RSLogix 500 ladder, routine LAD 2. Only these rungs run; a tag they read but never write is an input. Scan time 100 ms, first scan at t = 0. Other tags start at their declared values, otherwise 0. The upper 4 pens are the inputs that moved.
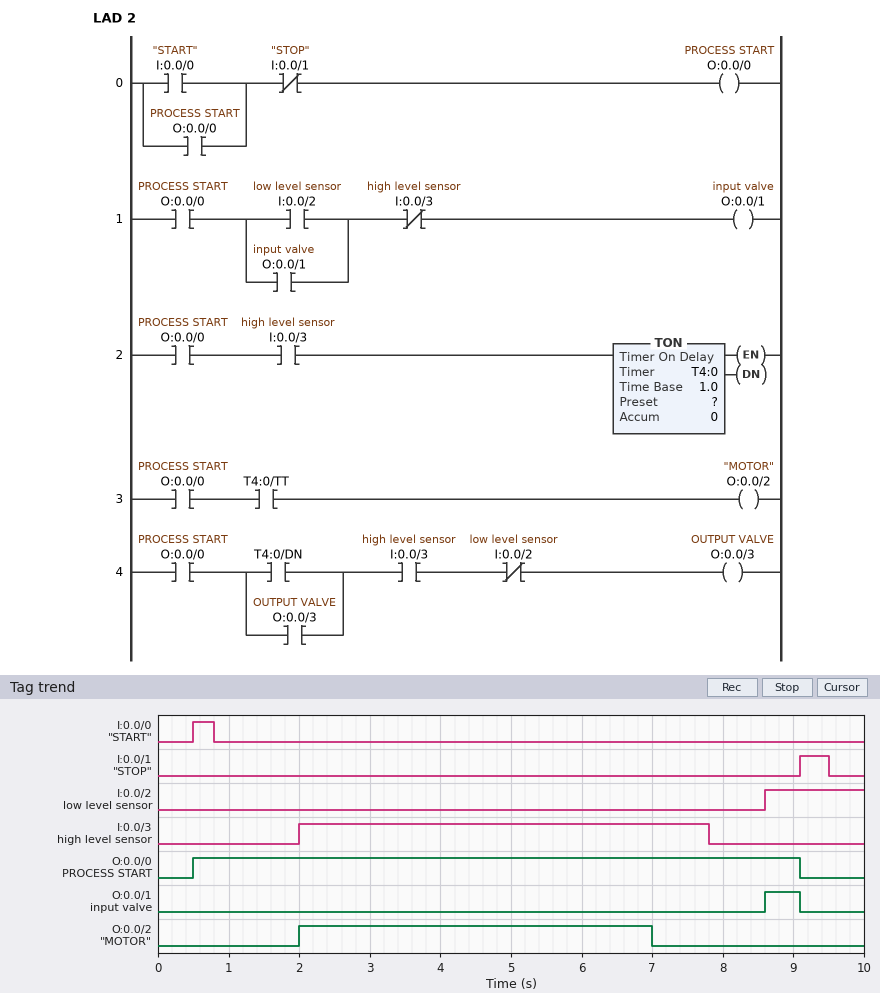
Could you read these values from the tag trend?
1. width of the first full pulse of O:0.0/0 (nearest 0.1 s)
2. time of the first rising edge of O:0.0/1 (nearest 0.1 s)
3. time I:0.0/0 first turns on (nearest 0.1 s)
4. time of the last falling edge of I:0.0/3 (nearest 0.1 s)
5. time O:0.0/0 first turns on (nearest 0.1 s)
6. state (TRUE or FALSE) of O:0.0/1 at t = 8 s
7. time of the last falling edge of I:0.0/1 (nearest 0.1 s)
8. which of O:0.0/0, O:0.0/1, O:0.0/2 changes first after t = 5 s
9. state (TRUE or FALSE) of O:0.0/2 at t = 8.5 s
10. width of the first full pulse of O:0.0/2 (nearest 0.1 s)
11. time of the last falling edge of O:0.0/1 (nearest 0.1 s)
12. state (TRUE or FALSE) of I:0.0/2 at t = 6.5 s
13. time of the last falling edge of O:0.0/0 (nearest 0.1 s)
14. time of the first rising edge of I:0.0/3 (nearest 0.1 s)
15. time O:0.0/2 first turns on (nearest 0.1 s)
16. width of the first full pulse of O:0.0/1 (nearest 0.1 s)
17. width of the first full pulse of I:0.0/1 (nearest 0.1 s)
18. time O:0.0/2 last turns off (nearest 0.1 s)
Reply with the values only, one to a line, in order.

8.6 s
8.6 s
0.5 s
7.8 s
0.5 s
FALSE
9.5 s
O:0.0/2
FALSE
5.0 s
9.1 s
FALSE
9.1 s
2.0 s
2.0 s
0.5 s
0.4 s
7.0 s
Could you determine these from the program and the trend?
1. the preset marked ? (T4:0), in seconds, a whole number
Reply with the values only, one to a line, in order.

5 s
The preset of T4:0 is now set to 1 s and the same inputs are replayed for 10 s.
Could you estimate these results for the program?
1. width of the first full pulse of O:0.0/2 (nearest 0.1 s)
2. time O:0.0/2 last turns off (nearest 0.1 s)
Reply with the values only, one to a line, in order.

1.0 s
3.0 s
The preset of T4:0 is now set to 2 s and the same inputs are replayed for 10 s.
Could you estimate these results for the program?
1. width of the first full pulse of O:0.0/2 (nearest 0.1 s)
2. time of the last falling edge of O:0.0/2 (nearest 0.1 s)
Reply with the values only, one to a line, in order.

2.0 s
4.0 s
